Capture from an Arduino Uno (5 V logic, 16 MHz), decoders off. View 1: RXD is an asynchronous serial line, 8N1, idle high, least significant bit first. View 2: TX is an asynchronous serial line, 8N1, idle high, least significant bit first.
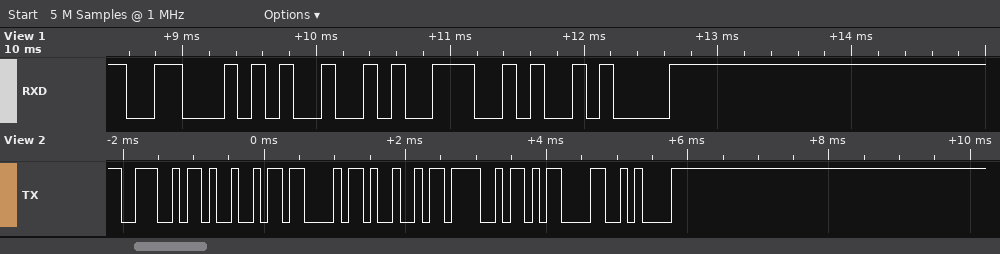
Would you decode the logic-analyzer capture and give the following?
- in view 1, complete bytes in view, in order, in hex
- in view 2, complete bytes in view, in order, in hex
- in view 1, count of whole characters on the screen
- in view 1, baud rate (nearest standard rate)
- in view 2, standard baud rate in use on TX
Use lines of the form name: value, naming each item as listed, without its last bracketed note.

in view 1, complete bytes in view, in order, in hex: 46 49 4E 0A
in view 2, complete bytes in view, in order, in hex: 0x4E 0x49 0x43 0x49 0x4F 0x0D 0x0A
in view 1, count of whole characters on the screen: 4
in view 1, baud rate: 9600 baud
in view 2, standard baud rate in use on TX: 9600 baud
